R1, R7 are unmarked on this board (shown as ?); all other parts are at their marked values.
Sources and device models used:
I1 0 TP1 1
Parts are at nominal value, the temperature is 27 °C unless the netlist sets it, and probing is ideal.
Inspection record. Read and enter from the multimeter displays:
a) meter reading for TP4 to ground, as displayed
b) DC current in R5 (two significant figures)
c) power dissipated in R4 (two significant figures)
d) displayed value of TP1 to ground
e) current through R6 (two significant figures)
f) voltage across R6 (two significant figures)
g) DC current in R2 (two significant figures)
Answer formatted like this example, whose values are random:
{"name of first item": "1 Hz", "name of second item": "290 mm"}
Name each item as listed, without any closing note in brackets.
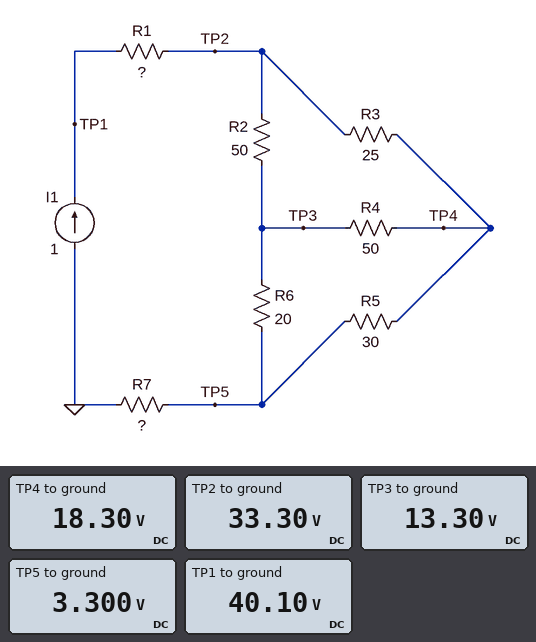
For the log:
{"meter reading for TP4 to ground, as displayed": "18.30 V", "DC current in R5": "500 mA", "power dissipated in R4": "500 mW", "displayed value of TP1 to ground": "40.10 V", "current through R6": "500 mA", "voltage across R6": "10 V", "DC current in R2": "400 mA"}
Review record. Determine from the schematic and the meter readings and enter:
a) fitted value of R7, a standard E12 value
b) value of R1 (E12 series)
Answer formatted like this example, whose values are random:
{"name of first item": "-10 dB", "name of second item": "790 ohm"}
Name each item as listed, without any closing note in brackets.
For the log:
{"fitted value of R7, a standard E12 value": "3.3 Ω", "value of R1": "6.8 Ω"}
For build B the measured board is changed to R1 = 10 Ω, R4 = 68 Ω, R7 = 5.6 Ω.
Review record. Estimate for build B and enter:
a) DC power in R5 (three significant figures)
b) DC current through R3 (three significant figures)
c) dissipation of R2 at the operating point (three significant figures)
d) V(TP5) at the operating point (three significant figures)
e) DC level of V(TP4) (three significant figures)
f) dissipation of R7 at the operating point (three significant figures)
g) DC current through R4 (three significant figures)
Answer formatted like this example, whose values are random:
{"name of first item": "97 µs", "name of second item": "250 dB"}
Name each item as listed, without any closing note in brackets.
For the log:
{"DC power in R5": "7.83 W", "DC current through R3": "593 mA", "dissipation of R2 at the operating point": "8.30 W", "V(TP5) at the operating point": "5.60 V", "DC level of V(TP4)": "20.9 V", "dissipation of R7 at the operating point": "5.60 W", "DC current through R4": "81.6 mA"}
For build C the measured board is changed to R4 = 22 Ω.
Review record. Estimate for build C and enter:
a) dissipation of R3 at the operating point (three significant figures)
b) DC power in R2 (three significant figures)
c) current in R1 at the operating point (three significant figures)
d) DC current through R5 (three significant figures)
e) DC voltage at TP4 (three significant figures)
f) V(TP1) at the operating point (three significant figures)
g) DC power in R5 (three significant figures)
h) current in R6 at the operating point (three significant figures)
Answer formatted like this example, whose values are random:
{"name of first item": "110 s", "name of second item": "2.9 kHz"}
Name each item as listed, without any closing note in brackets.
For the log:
{"dissipation of R3 at the operating point": "9.66 W", "DC power in R2": "7.16 W", "current in R1 at the operating point": "1.00 A", "DC current through R5": "468 mA", "DC voltage at TP4": "17.3 V", "V(TP1) at the operating point": "39.7 V", "DC power in R5": "6.56 W", "current in R6 at the operating point": "532 mA"}
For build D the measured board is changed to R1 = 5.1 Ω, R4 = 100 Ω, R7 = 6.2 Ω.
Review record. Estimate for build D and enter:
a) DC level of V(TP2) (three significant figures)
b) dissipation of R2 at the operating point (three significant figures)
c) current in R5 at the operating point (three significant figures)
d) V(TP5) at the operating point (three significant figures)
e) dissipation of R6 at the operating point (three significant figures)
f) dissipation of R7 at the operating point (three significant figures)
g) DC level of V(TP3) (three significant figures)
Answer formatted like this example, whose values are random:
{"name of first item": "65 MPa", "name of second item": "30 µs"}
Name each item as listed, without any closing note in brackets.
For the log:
{"DC level of V(TP2)": "36.5 V", "dissipation of R2 at the operating point": "8.63 W", "current in R5 at the operating point": "523 mA", "V(TP5) at the operating point": "6.20 V", "dissipation of R6 at the operating point": "4.55 W", "dissipation of R7 at the operating point": "6.20 W", "DC level of V(TP3)": "15.7 V"}
